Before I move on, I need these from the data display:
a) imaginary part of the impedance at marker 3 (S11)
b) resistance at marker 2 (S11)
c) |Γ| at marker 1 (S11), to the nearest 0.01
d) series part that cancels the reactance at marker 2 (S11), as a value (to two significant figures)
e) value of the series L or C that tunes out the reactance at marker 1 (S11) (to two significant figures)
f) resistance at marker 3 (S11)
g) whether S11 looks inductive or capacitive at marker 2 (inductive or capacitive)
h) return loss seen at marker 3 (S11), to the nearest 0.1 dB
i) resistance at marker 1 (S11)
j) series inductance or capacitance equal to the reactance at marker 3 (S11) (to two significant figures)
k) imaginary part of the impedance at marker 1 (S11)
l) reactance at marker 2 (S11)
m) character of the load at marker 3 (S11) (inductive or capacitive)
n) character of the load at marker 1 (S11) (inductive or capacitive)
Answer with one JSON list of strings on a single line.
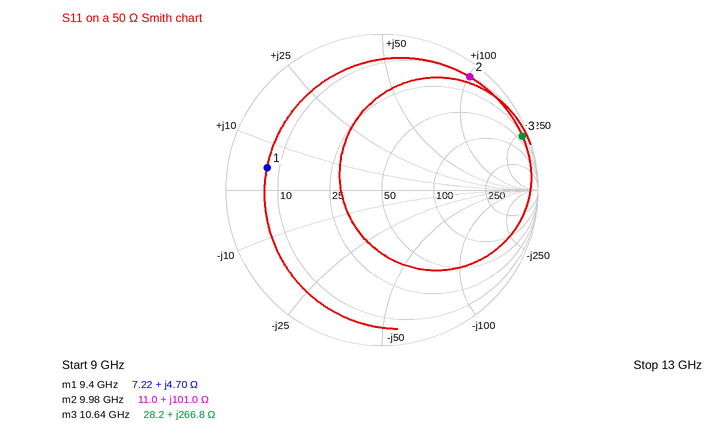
["+266.8 Ω", "11.0 Ω", "0.75", "160 fF", "3.6 pF", "28.2 Ω", "inductive", "0.3 dB", "7.22 Ω", "4.0 nH", "+4.70 Ω", "+101.0 Ω", "inductive", "inductive"]
